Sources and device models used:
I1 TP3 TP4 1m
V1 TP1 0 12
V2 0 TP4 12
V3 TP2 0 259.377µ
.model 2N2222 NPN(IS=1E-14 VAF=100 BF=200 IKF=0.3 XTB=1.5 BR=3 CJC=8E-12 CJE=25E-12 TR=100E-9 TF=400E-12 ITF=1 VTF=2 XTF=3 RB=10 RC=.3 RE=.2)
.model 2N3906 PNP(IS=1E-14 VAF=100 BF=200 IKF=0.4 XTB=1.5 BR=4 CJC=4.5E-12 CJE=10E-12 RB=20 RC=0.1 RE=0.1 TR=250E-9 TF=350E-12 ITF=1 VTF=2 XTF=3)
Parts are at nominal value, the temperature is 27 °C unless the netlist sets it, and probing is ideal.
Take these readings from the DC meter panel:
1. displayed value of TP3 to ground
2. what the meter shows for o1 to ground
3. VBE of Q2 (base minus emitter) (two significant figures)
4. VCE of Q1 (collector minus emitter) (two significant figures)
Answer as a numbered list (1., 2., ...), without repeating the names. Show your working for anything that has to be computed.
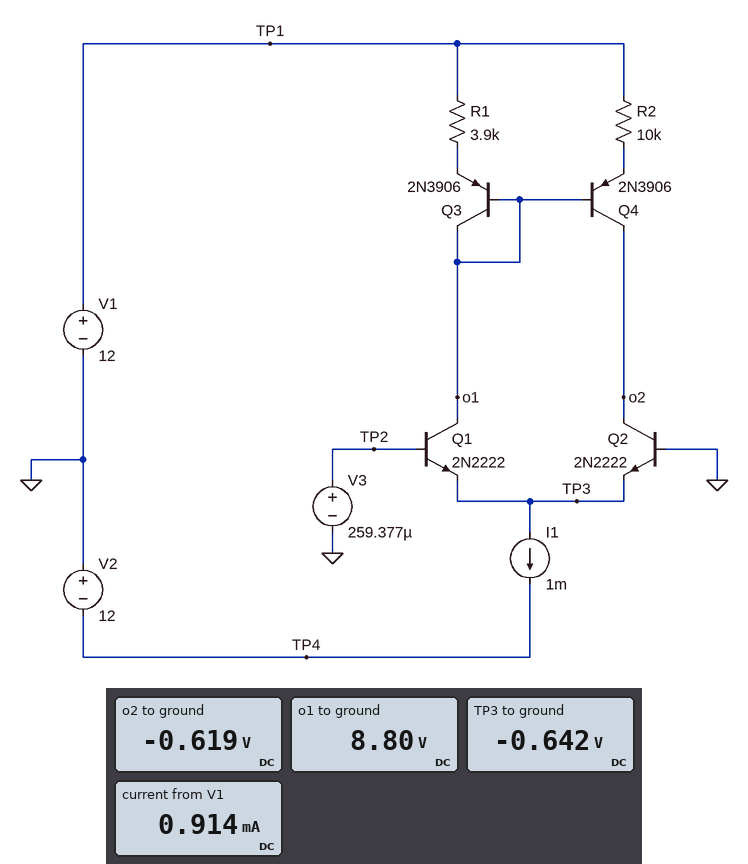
1. -0.642 V
2. 8.80 V
3. 0 V - (-642 mV) = 640 mV
4. 8.8 V - (-642 mV) = 9.4 V
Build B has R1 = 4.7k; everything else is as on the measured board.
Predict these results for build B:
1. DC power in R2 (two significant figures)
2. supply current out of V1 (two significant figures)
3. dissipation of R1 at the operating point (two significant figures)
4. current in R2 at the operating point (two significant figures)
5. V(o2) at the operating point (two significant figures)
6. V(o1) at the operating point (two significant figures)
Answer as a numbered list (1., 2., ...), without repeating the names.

1. 890 µW
2. 930 µA
3. 1.9 mW
4. 300 µA
5. -610 mV
6. 8.4 V
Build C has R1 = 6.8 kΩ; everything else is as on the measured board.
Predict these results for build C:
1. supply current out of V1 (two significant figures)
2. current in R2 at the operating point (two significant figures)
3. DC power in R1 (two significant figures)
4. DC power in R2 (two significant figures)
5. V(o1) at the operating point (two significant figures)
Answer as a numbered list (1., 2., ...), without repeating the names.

1. 960 µA
2. 390 µA
3. 2.2 mW
4. 1.5 mW
5. 7.5 V
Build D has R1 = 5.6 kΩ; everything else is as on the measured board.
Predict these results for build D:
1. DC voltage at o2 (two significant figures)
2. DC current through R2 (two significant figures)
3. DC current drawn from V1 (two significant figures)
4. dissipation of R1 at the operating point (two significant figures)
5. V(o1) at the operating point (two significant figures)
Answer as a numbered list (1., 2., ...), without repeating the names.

1. -610 mV
2. 340 µA
3. 940 µA
4. 2.0 mW
5. 8.0 V
